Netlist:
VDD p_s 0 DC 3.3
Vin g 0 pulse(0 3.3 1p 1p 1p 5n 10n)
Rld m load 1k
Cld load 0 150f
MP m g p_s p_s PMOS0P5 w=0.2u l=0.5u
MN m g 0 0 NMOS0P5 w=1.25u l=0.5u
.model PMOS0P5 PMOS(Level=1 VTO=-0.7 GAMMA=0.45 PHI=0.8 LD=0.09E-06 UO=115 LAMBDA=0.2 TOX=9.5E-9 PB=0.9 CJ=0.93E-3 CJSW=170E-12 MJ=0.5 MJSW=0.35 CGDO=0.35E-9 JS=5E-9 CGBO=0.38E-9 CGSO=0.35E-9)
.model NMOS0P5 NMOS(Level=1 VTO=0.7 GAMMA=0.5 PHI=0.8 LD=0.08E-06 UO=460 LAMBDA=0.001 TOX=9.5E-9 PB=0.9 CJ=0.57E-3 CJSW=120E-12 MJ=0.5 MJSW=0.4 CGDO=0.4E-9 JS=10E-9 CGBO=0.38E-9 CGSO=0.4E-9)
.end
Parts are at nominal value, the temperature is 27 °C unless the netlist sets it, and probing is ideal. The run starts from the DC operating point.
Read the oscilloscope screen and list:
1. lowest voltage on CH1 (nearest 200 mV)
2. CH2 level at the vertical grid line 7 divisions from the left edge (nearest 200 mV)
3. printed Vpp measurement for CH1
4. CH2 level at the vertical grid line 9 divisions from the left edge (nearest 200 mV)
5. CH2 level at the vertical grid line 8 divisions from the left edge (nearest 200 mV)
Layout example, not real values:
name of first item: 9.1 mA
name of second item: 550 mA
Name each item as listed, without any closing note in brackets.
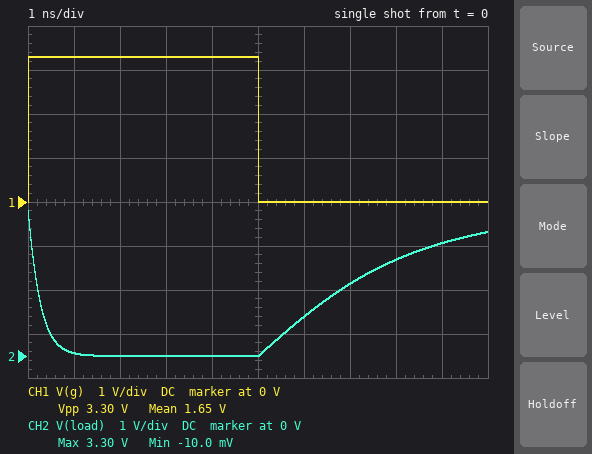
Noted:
lowest voltage on CH1: 0 V
CH2 level at the vertical grid line 7 divisions from the left edge: 1.6 V
printed Vpp measurement for CH1: 3.30 V
CH2 level at the vertical grid line 9 divisions from the left edge: 2.6 V
CH2 level at the vertical grid line 8 divisions from the left edge: 2.2 V
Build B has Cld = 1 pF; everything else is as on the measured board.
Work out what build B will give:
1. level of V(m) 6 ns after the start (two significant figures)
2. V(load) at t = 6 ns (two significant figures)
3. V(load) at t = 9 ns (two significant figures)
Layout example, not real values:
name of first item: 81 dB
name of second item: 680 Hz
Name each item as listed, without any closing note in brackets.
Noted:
level of V(m) 6 ns after the start: 450 mV
V(load) at t = 6 ns: 310 mV
V(load) at t = 9 ns: 710 mV
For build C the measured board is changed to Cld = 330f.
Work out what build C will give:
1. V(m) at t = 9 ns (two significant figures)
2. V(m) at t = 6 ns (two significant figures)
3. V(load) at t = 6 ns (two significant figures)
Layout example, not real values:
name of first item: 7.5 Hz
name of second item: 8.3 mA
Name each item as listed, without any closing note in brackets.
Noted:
V(m) at t = 9 ns: 1.6 V
V(m) at t = 6 ns: 560 mV
V(load) at t = 6 ns: 420 mV
